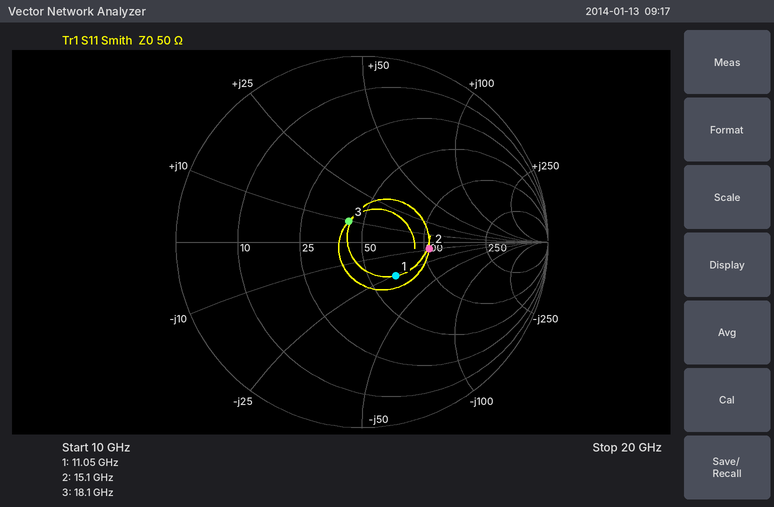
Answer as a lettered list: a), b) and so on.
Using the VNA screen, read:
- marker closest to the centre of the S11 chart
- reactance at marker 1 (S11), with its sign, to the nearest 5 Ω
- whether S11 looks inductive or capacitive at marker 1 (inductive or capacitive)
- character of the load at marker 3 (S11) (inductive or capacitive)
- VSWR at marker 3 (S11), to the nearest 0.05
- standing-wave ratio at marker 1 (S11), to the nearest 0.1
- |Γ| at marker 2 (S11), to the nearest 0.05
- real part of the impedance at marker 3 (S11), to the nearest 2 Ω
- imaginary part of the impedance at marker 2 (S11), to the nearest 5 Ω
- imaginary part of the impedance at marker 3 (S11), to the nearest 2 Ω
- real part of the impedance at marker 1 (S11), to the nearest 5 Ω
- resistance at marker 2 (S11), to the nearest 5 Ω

a) marker 3
b) -25 Ω
c) capacitive
d) inductive
e) 1.30
f) 1.7
g) 0.35
h) 42 Ω
i) -10 Ω
j) +10 Ω
k) 65 Ω
l) 105 Ω
